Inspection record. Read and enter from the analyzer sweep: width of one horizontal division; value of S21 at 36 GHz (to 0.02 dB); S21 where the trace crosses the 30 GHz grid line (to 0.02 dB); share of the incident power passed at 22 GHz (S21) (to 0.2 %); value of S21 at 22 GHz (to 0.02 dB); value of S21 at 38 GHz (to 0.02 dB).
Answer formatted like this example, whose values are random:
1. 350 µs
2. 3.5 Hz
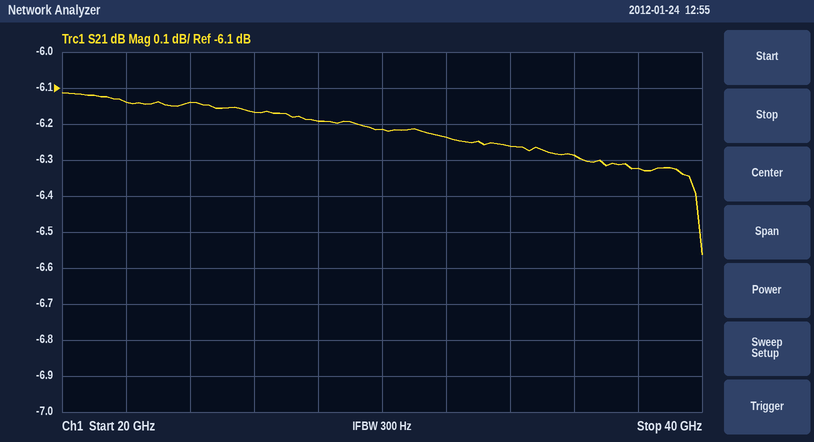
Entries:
1. 2 GHz
2. -6.28 dB
3. -6.22 dB
4. 24.4 %
5. -6.14 dB
6. -6.32 dB
